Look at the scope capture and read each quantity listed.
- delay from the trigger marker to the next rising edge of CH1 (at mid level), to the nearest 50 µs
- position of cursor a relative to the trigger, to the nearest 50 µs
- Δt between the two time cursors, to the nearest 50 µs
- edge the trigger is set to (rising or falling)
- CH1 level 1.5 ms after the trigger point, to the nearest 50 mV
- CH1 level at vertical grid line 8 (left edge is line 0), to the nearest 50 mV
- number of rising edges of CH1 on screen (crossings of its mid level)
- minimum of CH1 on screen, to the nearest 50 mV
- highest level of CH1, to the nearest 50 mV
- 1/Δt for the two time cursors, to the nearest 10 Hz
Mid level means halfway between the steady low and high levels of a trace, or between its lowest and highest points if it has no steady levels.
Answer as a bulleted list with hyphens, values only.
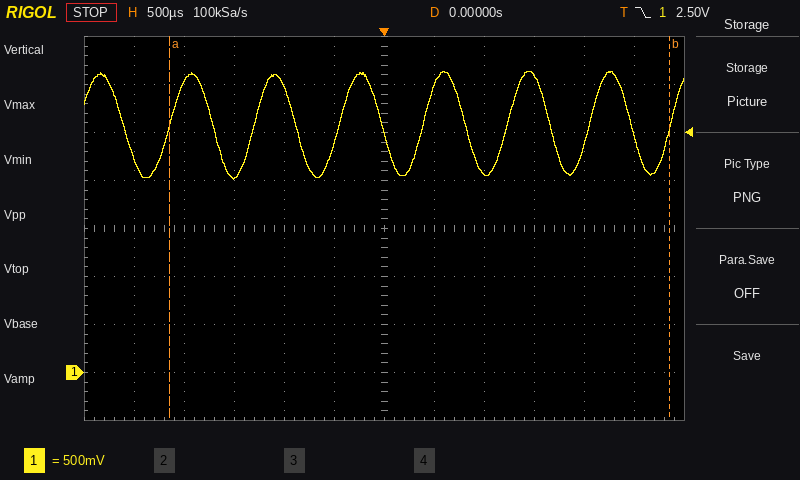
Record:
- 400 µs
- -2.15 ms
- 5.00 ms
- falling
- 3.10 V
- 2.10 V
- 7
- 2.00 V
- 3.15 V
- 200 Hz
